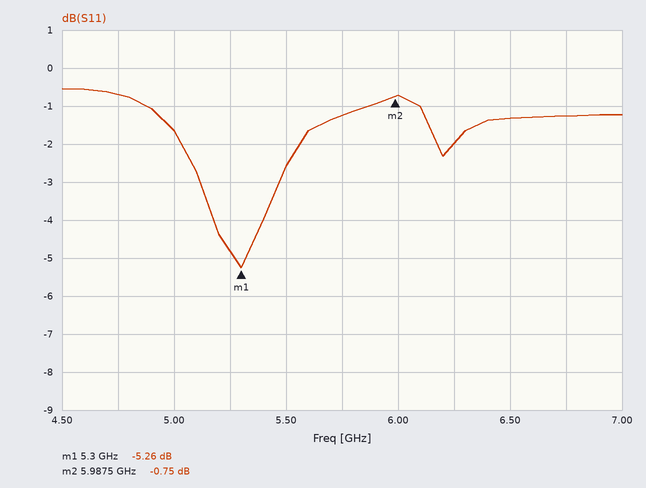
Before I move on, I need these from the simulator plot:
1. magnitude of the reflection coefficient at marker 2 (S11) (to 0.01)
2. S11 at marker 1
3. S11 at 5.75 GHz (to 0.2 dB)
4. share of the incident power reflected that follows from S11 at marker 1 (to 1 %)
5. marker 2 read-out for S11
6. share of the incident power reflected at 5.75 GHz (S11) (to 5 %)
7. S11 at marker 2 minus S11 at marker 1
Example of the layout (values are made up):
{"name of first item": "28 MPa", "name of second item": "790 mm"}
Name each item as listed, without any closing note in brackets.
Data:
{"magnitude of the reflection coefficient at marker 2 (S11)": "0.92", "S11 at marker 1": "-5.26 dB", "S11 at 5.75 GHz": "-1.2 dB", "share of the incident power reflected that follows from S11 at marker 1": "30 %", "marker 2 read-out for S11": "-0.75 dB", "share of the incident power reflected at 5.75 GHz (S11)": "75 %", "S11 at marker 2 minus S11 at marker 1": "4.51 dB"}
